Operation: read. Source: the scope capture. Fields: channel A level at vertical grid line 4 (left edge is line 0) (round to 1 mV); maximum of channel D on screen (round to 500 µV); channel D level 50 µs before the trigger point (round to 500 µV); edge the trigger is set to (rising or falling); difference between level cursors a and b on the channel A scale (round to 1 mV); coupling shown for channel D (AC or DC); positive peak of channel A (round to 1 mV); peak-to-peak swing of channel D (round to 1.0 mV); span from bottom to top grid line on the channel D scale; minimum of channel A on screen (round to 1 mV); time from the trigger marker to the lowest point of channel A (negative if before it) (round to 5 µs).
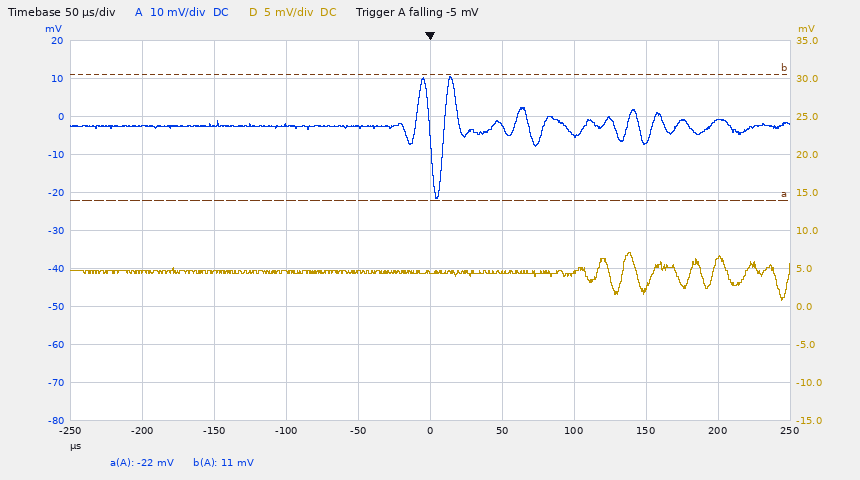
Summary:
-3 mV
7.0 mV
4.5 mV
falling
33 mV
DC
11 mV
6.0 mV
50 mV
-22 mV
+5 µs
